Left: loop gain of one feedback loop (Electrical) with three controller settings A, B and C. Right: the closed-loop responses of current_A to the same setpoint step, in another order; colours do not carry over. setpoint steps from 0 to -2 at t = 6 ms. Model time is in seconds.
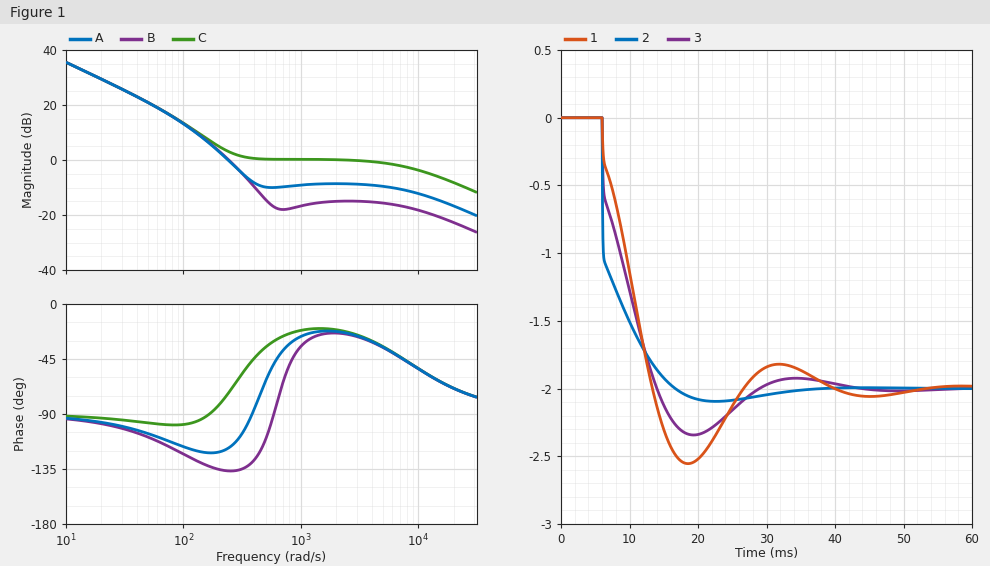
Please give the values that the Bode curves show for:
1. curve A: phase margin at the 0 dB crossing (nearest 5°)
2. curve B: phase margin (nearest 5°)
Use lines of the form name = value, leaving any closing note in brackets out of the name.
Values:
curve A: phase margin at the 0 dB crossing = 60°
curve B: phase margin = 45°
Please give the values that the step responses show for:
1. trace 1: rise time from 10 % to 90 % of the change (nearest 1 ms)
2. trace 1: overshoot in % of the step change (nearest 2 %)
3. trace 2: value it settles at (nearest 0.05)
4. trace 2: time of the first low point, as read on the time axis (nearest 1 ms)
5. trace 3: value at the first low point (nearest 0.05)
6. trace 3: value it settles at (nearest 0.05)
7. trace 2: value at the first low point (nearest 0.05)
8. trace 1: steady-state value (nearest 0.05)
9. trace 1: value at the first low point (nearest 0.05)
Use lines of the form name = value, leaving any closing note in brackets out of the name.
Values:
trace 1: rise time from 10 % to 90 % of the change = 6 ms
trace 1: overshoot in % of the step change = 28 %
trace 2: value it settles at = -2.00
trace 2: time of the first low point, as read on the time axis = 23 ms
trace 3: value at the first low point = -2.35
trace 3: value it settles at = -2.00
trace 2: value at the first low point = -2.10
trace 1: steady-state value = -2.00
trace 1: value at the first low point = -2.55
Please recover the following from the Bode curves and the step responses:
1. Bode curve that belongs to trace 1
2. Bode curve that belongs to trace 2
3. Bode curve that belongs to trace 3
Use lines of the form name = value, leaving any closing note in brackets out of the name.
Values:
Bode curve that belongs to trace 1 = B
Bode curve that belongs to trace 2 = C
Bode curve that belongs to trace 3 = A
